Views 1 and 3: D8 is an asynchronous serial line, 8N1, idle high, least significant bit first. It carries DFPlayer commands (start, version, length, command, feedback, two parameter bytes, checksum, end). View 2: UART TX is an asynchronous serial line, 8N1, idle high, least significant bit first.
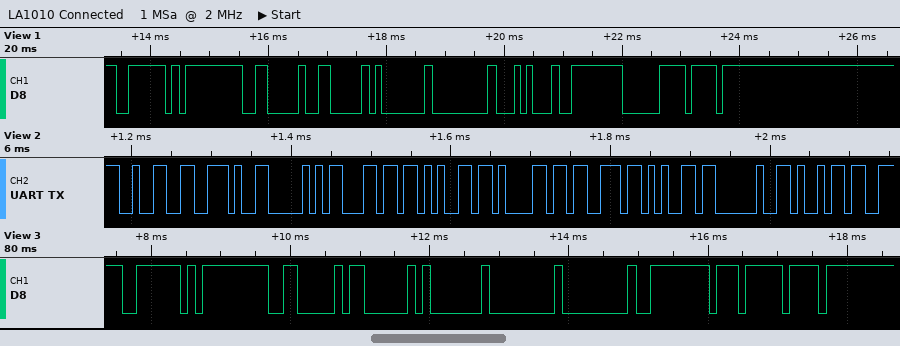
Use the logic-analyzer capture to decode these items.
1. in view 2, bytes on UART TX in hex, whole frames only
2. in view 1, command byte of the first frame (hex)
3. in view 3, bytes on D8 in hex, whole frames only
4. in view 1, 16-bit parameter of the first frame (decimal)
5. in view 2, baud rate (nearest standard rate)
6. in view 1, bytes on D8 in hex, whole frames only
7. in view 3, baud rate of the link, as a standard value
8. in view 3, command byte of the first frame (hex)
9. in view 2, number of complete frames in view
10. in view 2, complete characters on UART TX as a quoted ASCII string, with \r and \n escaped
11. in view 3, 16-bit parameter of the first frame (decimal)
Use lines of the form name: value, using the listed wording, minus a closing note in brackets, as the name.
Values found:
in view 2, bytes on UART TX in hex, whole frames only: 32 2E 50 6C 65 61 73 65 20 69
in view 1, command byte of the first frame: 0x06
in view 3, bytes on D8 in hex, whole frames only: 0x7E 0xFF 0x06 0x03 0x01 0x00 0x00 0xFE 0xF7 0xEF
in view 1, 16-bit parameter of the first frame: 20
in view 2, baud rate: 115200 baud
in view 1, bytes on D8 in hex, whole frames only: 0x7E 0xFF 0x06 0x06 0x01 0x00 0x14 0xFE 0xE0 0xEF
in view 3, baud rate of the link, as a standard value: 9600 baud
in view 3, command byte of the first frame: 0x03
in view 2, number of complete frames in view: 10
in view 2, complete characters on UART TX as a quoted ASCII string, with \r and \n escaped: "2.Please i"
in view 3, 16-bit parameter of the first frame: 0
